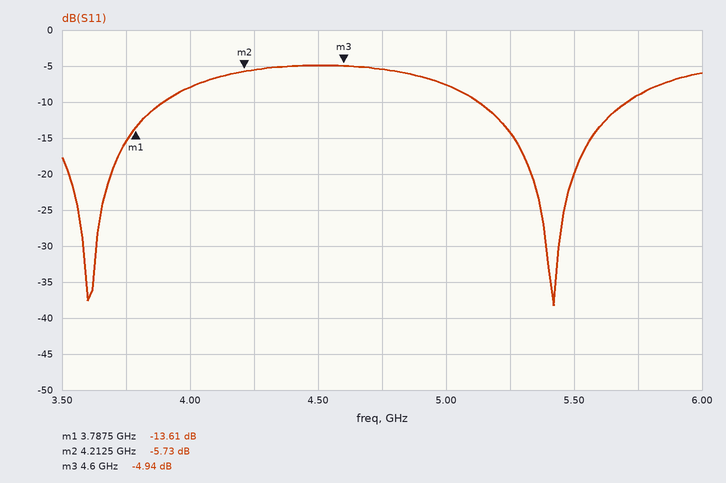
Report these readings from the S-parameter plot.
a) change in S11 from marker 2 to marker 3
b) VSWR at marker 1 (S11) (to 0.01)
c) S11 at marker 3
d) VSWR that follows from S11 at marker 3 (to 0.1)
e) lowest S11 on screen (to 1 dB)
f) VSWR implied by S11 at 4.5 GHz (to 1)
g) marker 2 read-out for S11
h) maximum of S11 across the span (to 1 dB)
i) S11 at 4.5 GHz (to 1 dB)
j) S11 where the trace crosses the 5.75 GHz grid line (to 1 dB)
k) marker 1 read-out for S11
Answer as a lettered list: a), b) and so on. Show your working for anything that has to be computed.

a) -4.94 − (-5.73) = 0.79 dB
b) (1 + 0.2087)/(1 − 0.2087) ≈ 1.53
c) -4.94 dB
d) (1 + 0.5662)/(1 − 0.5662) ≈ 3.6
e) -38 dB
f) |Γ| = 10^(-5/20) = 0.5623; VSWR = (1 + 0.5623)/(1 − 0.5623) ≈ 4
g) -5.73 dB
h) -5 dB
i) -5 dB
j) -9 dB
k) -13.61 dB
